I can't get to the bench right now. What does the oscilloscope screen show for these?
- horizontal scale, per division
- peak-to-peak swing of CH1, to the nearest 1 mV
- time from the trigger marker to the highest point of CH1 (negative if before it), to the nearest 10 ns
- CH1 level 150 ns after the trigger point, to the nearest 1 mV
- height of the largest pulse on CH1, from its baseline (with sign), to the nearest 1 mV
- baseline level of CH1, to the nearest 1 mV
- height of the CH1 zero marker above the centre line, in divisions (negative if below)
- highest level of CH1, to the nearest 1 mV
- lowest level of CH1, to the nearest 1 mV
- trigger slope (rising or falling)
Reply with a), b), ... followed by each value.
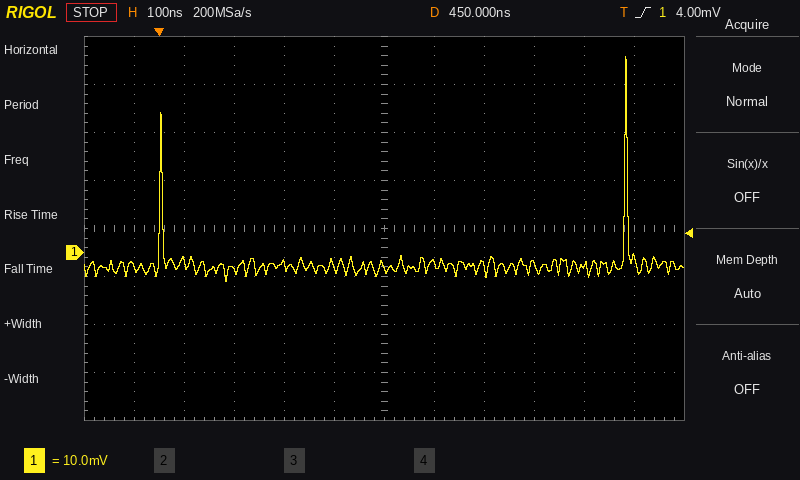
a) 100 ns
b) 47 mV
c) +930 ns
d) -4 mV
e) +44 mV
f) -3 mV
g) -0.5 div
h) 41 mV
i) -6 mV
j) rising
